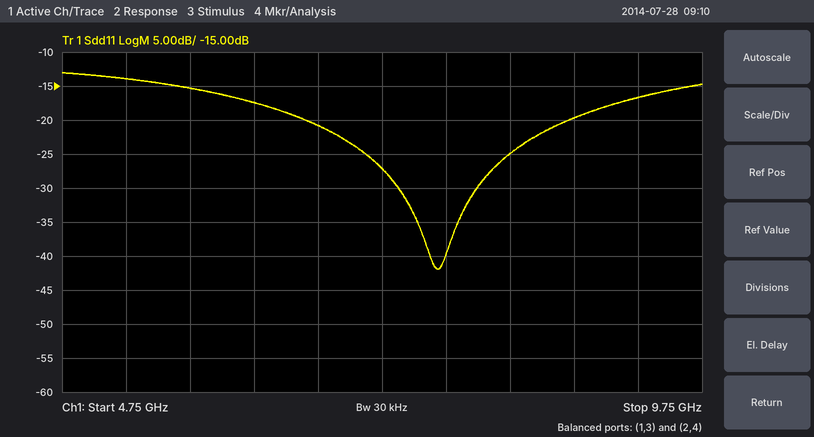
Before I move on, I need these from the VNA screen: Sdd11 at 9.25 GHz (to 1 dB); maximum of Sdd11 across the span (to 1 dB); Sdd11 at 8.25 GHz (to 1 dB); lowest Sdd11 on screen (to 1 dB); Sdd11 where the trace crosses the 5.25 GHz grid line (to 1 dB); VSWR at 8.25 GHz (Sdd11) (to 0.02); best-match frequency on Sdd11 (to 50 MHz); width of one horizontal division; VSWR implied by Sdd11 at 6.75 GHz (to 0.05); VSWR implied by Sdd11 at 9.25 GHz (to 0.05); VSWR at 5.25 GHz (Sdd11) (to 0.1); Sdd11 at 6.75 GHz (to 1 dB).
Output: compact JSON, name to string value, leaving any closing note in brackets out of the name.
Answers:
{"Sdd11 at 9.25 GHz": "-17 dB", "maximum of Sdd11 across the span": "-13 dB", "Sdd11 at 8.25 GHz": "-25 dB", "lowest Sdd11 on screen": "-42 dB", "Sdd11 where the trace crosses the 5.25 GHz grid line": "-14 dB", "VSWR at 8.25 GHz (Sdd11)": "1.12", "best-match frequency on Sdd11": "7.70 GHz", "width of one horizontal division": "500 MHz", "VSWR implied by Sdd11 at 6.75 GHz": "1.20", "VSWR implied by Sdd11 at 9.25 GHz": "1.35", "VSWR at 5.25 GHz (Sdd11)": "1.5", "Sdd11 at 6.75 GHz": "-21 dB"}
